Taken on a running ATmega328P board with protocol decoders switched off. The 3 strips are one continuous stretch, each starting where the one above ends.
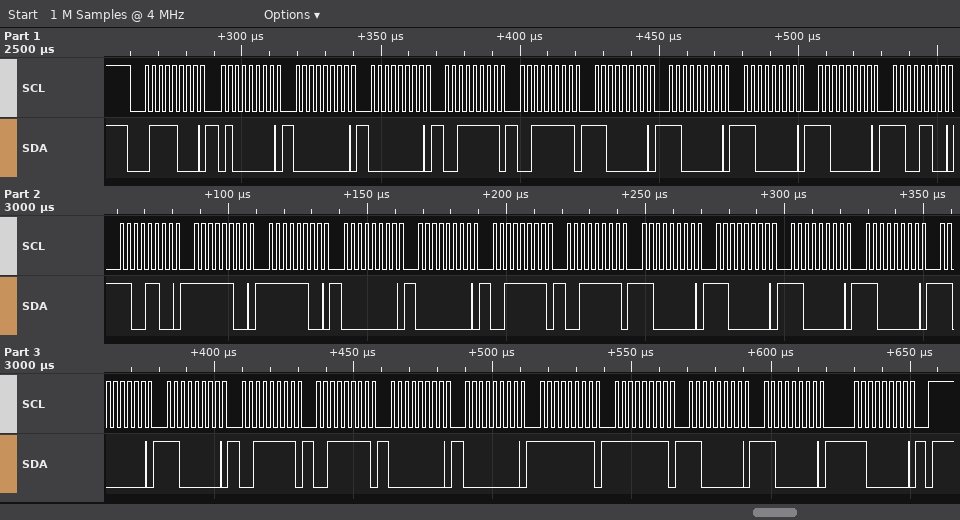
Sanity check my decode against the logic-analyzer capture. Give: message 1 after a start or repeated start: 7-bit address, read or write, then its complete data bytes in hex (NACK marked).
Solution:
0x3C write: 40 00 00 3F 3F C0 C0 C0 C0 CC CC FC FC 00 00 3F 3F C0 C0 C0 C0 C0 C0 3F 3F 00 00 FF FF C0 C0 C0
